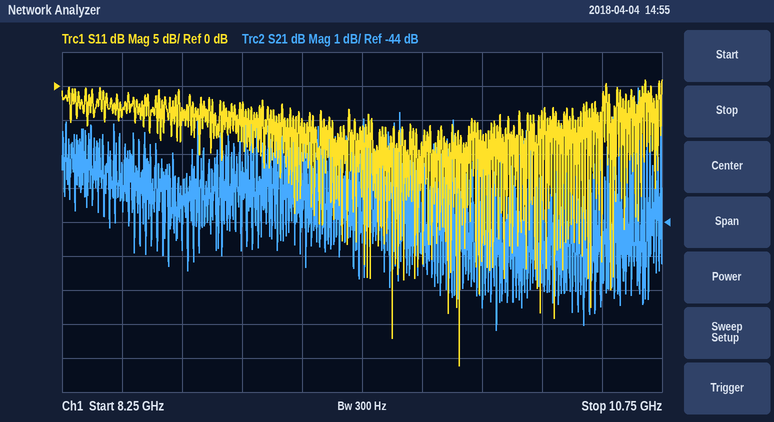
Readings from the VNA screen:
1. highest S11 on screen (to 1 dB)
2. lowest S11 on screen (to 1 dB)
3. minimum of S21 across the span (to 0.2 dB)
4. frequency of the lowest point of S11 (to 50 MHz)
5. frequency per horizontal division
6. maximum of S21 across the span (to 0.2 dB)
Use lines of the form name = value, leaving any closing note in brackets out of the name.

highest S11 on screen = 1 dB
lowest S11 on screen = -41 dB
minimum of S21 across the span = -47.2 dB
frequency of the lowest point of S11 = 9.90 GHz
frequency per horizontal division = 250 MHz
maximum of S21 across the span = -40.0 dB
